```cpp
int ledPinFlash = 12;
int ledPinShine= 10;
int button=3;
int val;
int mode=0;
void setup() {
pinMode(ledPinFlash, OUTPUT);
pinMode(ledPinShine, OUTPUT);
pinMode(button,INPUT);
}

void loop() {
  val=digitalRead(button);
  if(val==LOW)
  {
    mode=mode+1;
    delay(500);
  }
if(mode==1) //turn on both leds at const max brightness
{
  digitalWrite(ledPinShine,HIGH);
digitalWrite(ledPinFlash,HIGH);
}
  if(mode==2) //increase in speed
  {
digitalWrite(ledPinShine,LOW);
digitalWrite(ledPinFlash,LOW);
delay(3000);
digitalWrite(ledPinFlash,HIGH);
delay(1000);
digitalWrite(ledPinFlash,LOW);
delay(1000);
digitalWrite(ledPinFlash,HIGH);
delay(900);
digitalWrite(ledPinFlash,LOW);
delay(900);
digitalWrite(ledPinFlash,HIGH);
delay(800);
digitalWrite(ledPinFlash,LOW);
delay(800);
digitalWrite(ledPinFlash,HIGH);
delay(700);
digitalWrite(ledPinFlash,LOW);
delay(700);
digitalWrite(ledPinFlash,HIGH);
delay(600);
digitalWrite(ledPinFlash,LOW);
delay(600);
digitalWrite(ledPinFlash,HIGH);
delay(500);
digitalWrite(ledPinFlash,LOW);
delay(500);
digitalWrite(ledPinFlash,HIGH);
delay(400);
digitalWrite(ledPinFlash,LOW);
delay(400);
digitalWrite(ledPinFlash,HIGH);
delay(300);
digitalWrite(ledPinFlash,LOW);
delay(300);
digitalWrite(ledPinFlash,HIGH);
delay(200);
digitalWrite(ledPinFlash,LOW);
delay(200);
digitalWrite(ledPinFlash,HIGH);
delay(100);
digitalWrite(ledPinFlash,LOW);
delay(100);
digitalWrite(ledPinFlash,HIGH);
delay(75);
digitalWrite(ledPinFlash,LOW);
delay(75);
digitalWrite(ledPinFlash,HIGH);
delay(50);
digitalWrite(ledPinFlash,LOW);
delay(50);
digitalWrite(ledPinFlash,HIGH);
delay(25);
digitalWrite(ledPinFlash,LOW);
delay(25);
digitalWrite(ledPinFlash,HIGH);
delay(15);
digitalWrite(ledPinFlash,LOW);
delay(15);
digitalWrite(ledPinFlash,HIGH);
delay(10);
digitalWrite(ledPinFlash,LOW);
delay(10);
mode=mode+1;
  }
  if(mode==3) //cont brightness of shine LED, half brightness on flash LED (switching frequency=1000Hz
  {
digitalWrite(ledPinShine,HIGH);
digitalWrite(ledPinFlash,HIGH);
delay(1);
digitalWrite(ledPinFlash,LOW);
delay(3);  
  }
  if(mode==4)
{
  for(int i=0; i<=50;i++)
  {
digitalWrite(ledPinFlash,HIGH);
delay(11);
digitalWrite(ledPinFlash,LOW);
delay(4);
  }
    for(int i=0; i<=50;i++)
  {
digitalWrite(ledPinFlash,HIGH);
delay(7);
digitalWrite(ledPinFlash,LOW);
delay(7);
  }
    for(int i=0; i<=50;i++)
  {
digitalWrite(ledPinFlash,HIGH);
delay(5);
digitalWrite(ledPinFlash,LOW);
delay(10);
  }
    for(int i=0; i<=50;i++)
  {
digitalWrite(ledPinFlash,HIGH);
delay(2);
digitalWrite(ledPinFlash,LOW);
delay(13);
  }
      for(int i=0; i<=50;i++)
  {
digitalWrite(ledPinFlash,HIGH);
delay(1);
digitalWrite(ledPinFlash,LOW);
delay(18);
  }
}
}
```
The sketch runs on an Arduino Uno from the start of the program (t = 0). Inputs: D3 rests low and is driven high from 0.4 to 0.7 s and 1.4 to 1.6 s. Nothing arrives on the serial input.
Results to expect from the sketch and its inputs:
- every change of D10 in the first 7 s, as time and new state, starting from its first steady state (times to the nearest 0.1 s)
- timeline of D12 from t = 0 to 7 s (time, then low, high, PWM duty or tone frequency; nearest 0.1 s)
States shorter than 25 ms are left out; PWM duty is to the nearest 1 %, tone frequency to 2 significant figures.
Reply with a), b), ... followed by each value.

a) 0 s low; 0.5 s high; 1.2 s low
b) 0 s low; 0.5 s high; 1.2 s low; 4.2 s high; 5.2 s low; 6.2 s high
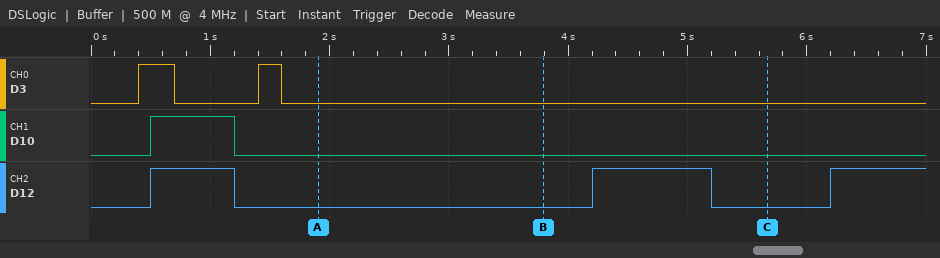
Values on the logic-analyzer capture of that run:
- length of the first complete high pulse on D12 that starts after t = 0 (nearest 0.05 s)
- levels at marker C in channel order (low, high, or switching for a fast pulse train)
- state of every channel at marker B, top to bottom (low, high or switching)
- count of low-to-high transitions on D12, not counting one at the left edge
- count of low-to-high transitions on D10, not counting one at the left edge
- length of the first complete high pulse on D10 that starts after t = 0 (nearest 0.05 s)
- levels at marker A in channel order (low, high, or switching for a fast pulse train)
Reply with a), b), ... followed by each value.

a) 0.70 s
b) D3 low, D10 low, D12 low
c) D3 low, D10 low, D12 low
d) 3
e) 1
f) 0.70 s
g) D3 low, D10 low, D12 low
